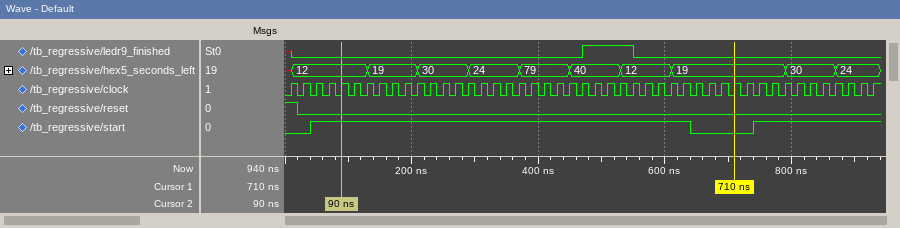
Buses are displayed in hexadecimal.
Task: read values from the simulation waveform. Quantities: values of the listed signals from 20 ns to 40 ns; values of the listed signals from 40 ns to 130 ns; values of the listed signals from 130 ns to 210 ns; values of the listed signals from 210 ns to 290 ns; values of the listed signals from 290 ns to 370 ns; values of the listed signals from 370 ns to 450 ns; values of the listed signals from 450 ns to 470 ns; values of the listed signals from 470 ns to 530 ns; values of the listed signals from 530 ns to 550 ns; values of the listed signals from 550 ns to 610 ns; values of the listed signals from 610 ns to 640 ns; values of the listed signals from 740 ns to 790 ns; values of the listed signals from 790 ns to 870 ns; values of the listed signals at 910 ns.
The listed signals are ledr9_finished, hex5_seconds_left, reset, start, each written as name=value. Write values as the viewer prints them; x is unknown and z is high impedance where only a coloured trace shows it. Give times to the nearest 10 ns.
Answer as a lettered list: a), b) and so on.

a) ledr9_finished=0, hex5_seconds_left=12, reset=0, start=0
b) ledr9_finished=0, hex5_seconds_left=12, reset=0, start=1
c) ledr9_finished=0, hex5_seconds_left=19, reset=0, start=1
d) ledr9_finished=0, hex5_seconds_left=30, reset=0, start=1
e) ledr9_finished=0, hex5_seconds_left=24, reset=0, start=1
f) ledr9_finished=0, hex5_seconds_left=79, reset=0, start=1
g) ledr9_finished=0, hex5_seconds_left=40, reset=0, start=1
h) ledr9_finished=1, hex5_seconds_left=40, reset=0, start=1
i) ledr9_finished=1, hex5_seconds_left=12, reset=0, start=1
j) ledr9_finished=0, hex5_seconds_left=12, reset=0, start=1
k) ledr9_finished=0, hex5_seconds_left=19, reset=0, start=1
l) ledr9_finished=0, hex5_seconds_left=19, reset=0, start=1
m) ledr9_finished=0, hex5_seconds_left=30, reset=0, start=1
n) ledr9_finished=0, hex5_seconds_left=24, reset=0, start=1
